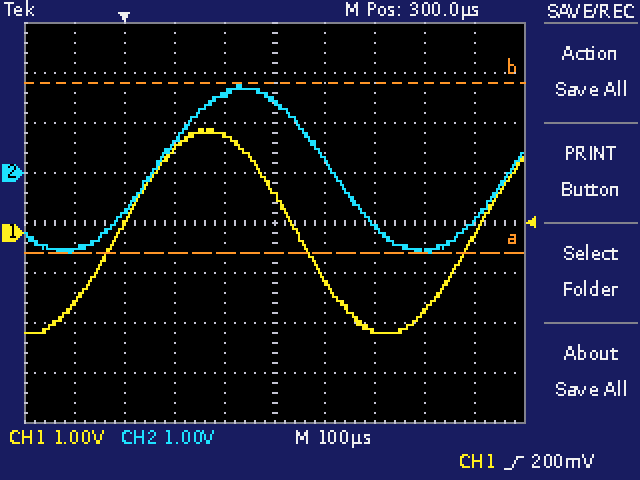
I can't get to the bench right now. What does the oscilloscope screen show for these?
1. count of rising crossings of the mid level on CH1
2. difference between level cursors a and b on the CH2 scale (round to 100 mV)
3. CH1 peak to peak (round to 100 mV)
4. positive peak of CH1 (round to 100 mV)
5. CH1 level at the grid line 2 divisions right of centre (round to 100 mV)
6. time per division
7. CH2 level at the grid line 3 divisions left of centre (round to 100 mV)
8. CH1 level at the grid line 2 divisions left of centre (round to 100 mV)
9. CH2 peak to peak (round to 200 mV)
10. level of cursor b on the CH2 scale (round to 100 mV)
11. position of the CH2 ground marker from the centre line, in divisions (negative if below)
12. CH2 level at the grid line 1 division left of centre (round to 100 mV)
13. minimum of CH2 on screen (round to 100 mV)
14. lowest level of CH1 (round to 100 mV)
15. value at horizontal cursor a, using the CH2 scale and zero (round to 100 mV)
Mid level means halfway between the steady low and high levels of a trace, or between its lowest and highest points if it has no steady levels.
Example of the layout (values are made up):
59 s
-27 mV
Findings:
2
3.4 V
4.1 V
2.1 V
-2.0 V
100 µs
-800 mV
1.7 V
3.4 V
1.8 V
+1.0 div
1.6 V
-1.6 V
-2.0 V
-1.6 V
